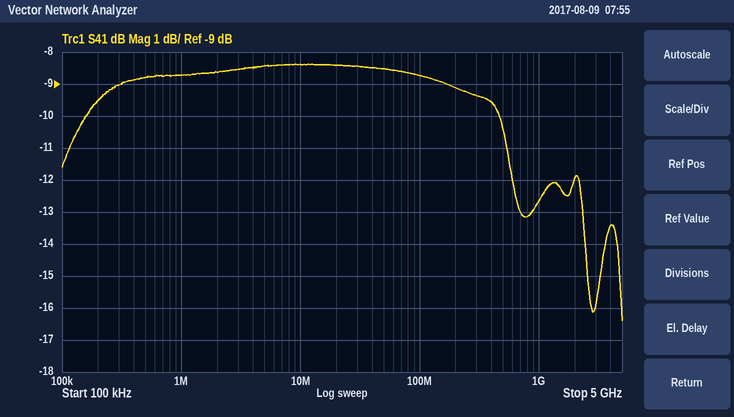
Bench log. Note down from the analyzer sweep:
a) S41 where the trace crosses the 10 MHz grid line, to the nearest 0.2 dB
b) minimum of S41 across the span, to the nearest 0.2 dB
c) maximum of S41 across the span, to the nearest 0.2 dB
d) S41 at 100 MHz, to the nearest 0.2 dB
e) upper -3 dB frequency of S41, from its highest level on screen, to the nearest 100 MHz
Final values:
-8.4 dB
-16.4 dB
-8.4 dB
-8.8 dB
600 MHz
